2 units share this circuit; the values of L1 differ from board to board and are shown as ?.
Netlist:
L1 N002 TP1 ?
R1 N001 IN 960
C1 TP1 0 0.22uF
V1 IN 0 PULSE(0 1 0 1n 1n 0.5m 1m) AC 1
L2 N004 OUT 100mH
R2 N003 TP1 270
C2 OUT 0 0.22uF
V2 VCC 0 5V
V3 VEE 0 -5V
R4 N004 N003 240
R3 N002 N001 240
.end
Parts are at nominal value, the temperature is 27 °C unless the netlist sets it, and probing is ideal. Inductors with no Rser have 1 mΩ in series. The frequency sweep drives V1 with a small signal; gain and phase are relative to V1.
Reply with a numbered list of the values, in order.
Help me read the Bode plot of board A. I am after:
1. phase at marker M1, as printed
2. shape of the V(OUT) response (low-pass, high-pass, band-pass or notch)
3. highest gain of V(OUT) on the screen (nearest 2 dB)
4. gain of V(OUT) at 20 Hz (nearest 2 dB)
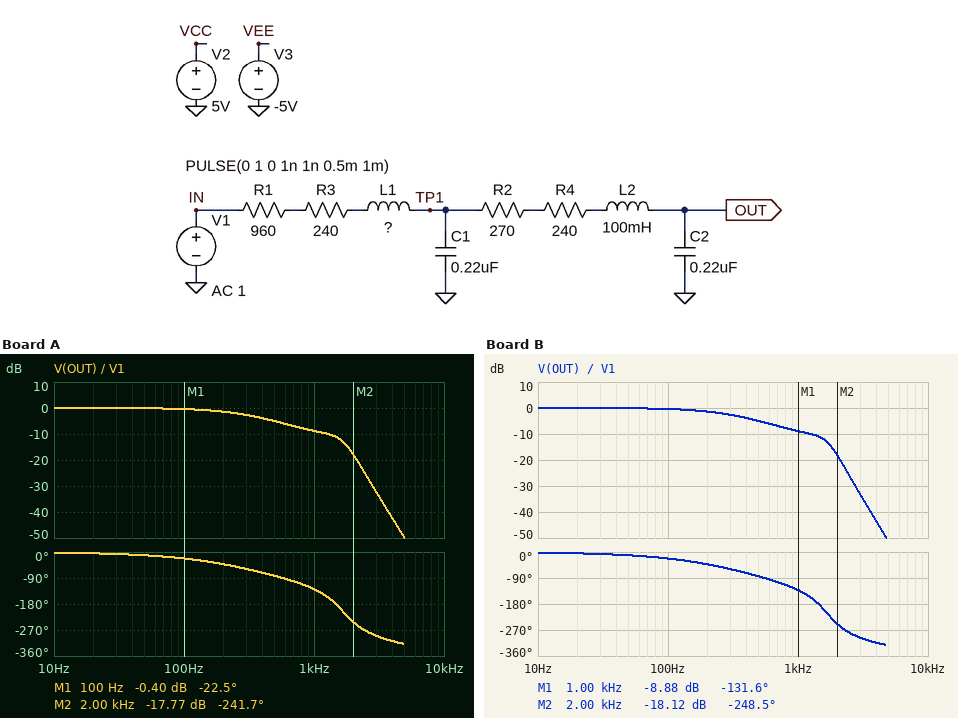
1. -22.5 deg
2. low-pass
3. 0 dB
4. 0 dB
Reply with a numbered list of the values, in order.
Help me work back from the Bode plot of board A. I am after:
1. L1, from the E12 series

1. 68 mH
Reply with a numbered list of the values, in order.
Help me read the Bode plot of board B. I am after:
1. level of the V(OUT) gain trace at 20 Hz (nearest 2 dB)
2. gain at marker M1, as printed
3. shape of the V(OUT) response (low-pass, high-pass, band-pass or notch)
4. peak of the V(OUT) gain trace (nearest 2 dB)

1. 0 dB
2. -8.88 dB
3. low-pass
4. 0 dB
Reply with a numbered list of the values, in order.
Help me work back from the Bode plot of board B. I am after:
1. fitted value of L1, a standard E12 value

1. 82 mH
